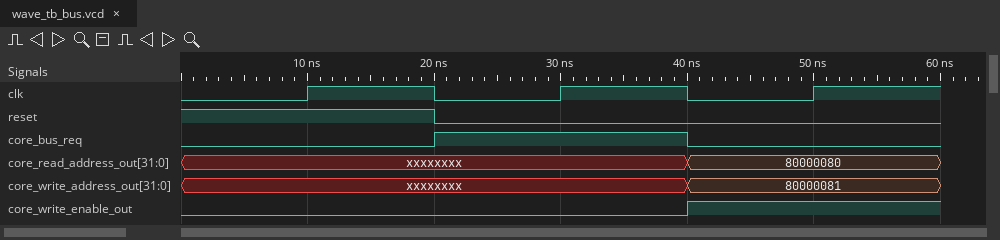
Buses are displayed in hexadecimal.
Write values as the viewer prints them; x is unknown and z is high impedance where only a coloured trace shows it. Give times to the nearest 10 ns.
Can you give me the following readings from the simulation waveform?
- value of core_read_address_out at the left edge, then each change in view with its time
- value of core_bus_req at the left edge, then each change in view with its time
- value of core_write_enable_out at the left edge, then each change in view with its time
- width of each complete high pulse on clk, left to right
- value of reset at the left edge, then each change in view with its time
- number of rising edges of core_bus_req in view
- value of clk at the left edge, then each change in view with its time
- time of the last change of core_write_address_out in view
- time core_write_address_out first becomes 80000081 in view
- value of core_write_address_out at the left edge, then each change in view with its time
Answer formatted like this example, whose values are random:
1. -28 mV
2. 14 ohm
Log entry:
1. xxxxxxxx, 80000080 at 40 ns
2. 0, 1 at 20 ns, 0 at 40 ns
3. 0, 1 at 40 ns
4. 10 ns, 10 ns
5. 1, 0 at 20 ns
6. 1
7. 0, 1 at 10 ns, 0 at 20 ns, 1 at 30 ns, 0 at 40 ns, 1 at 50 ns
8. 40 ns
9. 40 ns
10. xxxxxxxx, 80000081 at 40 ns
